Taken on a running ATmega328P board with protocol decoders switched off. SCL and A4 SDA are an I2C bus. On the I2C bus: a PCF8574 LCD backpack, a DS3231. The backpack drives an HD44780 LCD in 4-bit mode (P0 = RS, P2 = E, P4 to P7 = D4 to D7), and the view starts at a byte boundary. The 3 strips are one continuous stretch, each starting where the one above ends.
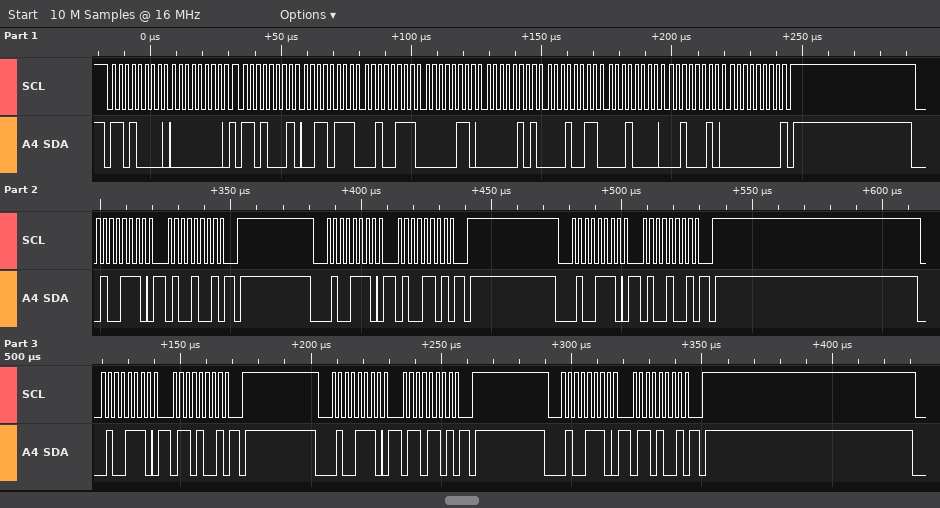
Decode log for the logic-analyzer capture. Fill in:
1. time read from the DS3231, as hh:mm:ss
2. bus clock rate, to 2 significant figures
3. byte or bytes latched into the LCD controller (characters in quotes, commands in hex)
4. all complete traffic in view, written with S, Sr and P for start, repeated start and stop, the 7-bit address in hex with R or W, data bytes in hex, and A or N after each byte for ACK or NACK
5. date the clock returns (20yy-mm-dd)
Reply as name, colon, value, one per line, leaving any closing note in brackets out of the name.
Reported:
time read from the DS3231, as hh:mm:ss: 06:27:37
bus clock rate, to 2 significant figures: 400 kHz
byte or bytes latched into the LCD controller: 'F'
all complete traffic in view, written with S, Sr and P for start, repeated start and stop, the 7-bit address in hex with R or W, data bytes in hex, and A or N after each byte for ACK or NACK: S 68W A 00 A Sr 68R A 37 A 27 A 06 A 05 A 13 A 10 A 22 A 00 N P S 27W A 49 A P S 27W A 4D A P S 27W A 49 A P S 27W A 69 A P S 27W A 6D A P S 27W A 69 A P
date the clock returns: 2022-10-13
